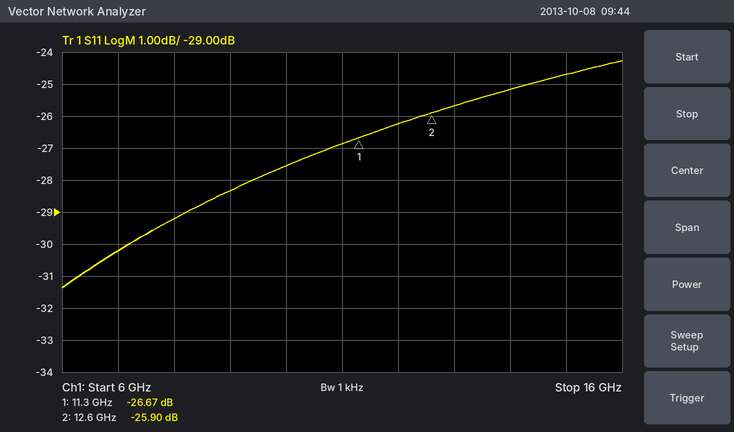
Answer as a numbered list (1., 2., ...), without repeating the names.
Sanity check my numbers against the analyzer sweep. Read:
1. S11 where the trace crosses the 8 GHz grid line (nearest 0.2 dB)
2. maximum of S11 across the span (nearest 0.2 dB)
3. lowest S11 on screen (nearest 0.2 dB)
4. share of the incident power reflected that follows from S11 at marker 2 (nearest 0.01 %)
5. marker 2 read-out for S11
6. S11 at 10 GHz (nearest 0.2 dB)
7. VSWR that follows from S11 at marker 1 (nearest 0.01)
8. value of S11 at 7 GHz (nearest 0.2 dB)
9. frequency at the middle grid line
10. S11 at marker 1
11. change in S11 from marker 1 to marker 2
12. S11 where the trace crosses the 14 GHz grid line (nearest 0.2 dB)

1. -29.2 dB
2. -24.2 dB
3. -31.4 dB
4. 0.26 %
5. -25.90 dB
6. -27.6 dB
7. 1.10
8. -30.2 dB
9. 11 GHz
10. -26.67 dB
11. 0.77 dB
12. -25.2 dB
